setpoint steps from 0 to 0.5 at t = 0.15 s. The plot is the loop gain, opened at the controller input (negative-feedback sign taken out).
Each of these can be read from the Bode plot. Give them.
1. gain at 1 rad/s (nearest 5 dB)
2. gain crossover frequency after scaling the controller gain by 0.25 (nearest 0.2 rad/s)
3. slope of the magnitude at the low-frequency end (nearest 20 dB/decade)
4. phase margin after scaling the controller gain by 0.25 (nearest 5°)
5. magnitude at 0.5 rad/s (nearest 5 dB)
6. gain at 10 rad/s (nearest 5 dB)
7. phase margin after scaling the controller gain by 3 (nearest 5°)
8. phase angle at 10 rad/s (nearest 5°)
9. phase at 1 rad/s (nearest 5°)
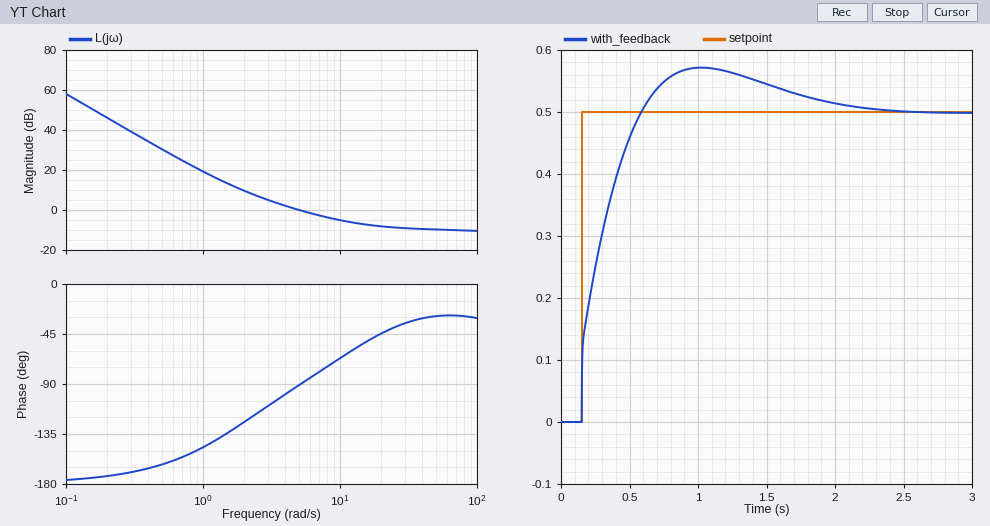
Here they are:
20 dB
1.6 rad/s
-40 dB/decade
50°
30 dB
-5 dB
150°
-65°
-145°
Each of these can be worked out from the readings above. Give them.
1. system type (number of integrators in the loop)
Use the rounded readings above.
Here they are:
2
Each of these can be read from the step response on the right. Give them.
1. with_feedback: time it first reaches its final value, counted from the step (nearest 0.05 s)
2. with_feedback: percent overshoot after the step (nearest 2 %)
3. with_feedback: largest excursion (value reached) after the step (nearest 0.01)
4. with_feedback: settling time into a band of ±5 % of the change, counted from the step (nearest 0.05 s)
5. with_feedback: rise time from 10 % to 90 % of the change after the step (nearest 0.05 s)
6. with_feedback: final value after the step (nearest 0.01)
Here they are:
0.45 s
14 %
0.57
1.65 s
0.35 s
0.50
